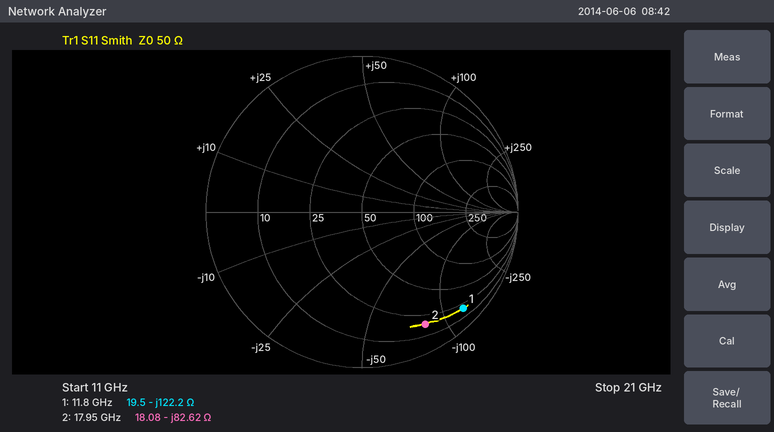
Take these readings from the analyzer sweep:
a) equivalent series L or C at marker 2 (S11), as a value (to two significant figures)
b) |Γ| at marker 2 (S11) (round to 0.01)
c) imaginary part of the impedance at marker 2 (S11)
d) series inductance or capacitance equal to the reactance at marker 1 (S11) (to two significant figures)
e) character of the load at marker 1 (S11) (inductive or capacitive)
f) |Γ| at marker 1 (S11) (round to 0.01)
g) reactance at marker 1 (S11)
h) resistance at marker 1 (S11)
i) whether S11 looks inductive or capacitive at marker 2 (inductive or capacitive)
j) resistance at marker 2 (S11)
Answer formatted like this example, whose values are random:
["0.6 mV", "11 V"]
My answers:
["110 fF", "0.83", "-82.62 Ω", "110 fF", "capacitive", "0.90", "-122.2 Ω", "19.5 Ω", "capacitive", "18.08 Ω"]
